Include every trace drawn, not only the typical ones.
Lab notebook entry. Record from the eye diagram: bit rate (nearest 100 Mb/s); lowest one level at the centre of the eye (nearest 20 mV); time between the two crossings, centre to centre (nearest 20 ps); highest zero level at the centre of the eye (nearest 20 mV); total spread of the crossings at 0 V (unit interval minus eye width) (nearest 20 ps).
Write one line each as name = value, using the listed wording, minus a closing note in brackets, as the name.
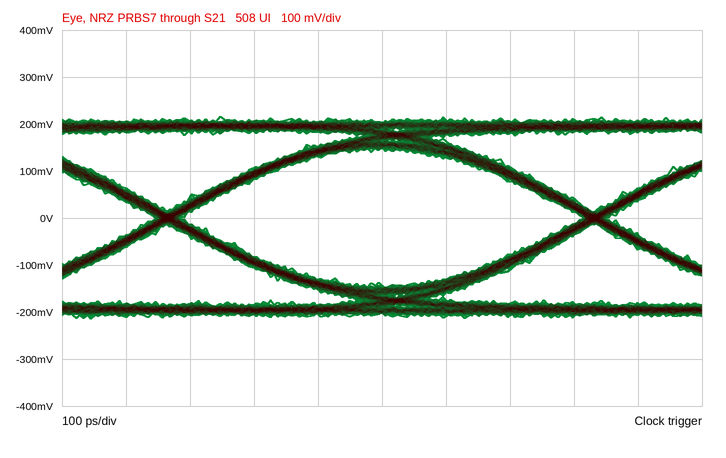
bit rate = 1.5 Gb/s
lowest one level at the centre of the eye = 140 mV
time between the two crossings, centre to centre = 660 ps
highest zero level at the centre of the eye = -140 mV
total spread of the crossings at 0 V (unit interval minus eye width) = 40 ps
